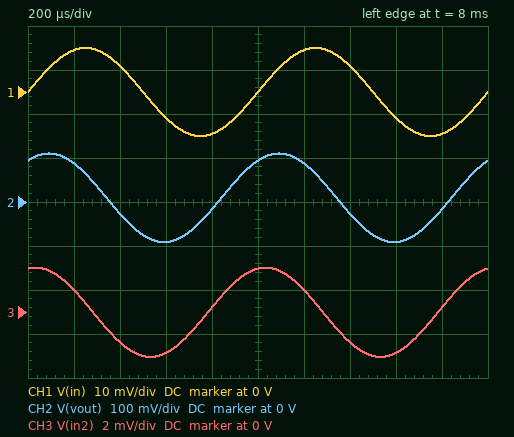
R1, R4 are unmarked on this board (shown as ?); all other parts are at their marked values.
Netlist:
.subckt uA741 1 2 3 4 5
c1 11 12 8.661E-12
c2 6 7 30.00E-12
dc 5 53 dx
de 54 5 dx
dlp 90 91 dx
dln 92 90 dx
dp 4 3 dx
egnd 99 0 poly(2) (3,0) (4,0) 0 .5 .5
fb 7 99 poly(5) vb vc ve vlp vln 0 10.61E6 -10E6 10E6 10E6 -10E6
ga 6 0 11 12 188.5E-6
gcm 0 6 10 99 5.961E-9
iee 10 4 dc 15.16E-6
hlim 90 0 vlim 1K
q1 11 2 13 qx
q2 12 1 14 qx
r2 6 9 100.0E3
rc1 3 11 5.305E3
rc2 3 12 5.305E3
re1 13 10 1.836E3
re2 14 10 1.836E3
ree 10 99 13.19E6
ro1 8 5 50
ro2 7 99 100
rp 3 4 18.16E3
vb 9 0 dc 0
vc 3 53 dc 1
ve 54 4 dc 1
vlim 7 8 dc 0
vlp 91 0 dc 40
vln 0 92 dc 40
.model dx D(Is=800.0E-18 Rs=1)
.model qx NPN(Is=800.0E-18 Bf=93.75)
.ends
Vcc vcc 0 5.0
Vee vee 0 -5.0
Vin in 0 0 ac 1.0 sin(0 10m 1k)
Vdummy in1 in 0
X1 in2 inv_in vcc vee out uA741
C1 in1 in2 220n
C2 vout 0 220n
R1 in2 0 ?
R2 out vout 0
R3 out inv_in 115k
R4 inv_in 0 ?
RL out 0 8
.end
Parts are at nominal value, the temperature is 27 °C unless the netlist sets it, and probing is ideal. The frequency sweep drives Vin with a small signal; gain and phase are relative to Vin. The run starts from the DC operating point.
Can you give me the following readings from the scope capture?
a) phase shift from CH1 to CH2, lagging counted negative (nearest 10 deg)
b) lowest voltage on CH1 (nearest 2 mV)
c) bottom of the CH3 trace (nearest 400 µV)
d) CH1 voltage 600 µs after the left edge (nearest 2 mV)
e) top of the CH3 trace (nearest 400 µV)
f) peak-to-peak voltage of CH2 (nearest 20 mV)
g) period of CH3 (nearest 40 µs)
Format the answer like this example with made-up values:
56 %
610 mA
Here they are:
60 deg
-10 mV
-2.0 mV
-6 mV
2.0 mV
200 mV
1.00 ms
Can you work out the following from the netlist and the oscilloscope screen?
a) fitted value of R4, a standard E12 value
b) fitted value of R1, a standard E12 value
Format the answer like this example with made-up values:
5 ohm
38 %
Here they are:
2.2 kΩ
150 Ω
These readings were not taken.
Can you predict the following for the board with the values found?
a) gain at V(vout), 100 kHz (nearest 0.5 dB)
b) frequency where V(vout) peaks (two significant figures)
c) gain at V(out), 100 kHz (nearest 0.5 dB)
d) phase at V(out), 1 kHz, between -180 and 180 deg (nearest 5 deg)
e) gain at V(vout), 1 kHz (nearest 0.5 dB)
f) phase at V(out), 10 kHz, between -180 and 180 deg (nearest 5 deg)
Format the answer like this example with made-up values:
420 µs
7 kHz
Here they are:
0 dB
3.6 kHz
0 dB
55 deg
20.0 dB
-55 deg
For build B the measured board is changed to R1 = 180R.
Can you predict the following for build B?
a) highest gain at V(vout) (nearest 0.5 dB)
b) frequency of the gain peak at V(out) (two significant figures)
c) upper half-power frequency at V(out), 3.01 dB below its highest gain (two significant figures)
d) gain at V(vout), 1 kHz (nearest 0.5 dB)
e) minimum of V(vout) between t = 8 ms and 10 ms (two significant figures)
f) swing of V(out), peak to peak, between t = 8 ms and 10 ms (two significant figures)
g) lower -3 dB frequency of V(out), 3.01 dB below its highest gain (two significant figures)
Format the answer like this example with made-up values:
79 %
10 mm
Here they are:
26.5 dB
3.3 kHz
8.0 kHz
21.5 dB
-110 mV
240 mV
1.3 kHz
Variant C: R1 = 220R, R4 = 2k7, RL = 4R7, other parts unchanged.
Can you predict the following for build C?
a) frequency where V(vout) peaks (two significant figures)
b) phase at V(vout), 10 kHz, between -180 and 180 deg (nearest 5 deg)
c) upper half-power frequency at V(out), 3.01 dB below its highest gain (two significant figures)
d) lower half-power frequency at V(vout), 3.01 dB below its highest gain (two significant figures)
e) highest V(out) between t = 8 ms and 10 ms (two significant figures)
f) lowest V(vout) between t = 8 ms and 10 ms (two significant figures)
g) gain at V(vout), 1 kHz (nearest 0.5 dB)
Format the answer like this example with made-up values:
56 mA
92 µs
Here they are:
2.6 kHz
-65 deg
6.3 kHz
1.0 kHz
120 mV
-100 mV
21.0 dB
